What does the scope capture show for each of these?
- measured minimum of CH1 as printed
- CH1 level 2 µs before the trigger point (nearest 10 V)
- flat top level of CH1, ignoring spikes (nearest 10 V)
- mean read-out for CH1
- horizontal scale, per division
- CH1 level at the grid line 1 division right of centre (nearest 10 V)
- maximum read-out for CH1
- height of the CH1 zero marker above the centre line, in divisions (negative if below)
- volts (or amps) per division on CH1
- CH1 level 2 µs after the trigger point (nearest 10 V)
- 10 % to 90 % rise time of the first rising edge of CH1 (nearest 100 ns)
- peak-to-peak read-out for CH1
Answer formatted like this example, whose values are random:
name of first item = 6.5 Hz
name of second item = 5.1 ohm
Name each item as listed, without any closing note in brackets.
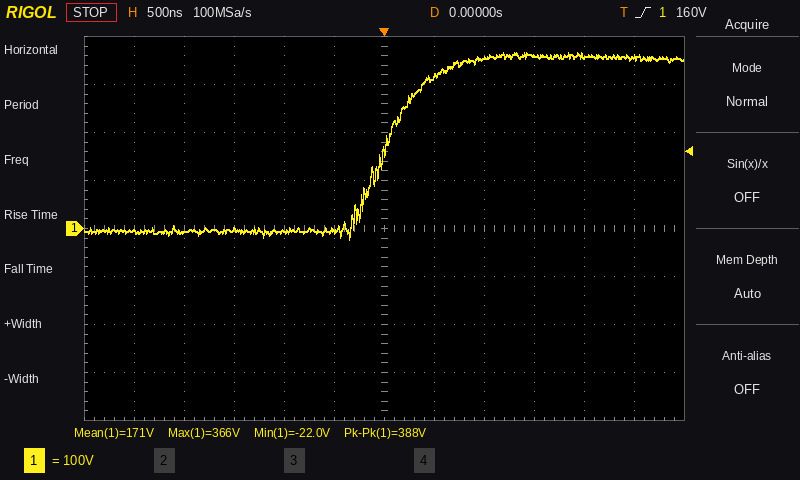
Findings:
measured minimum of CH1 as printed = -22.0 V
CH1 level 2 µs before the trigger point = -10 V
flat top level of CH1, ignoring spikes = 360 V
mean read-out for CH1 = 171 V
horizontal scale, per division = 500 ns
CH1 level at the grid line 1 division right of centre = 320 V
maximum read-out for CH1 = 366 V
height of the CH1 zero marker above the centre line, in divisions = 0.0 div
volts (or amps) per division on CH1 = 100 V
CH1 level 2 µs after the trigger point = 360 V
10 % to 90 % rise time of the first rising edge of CH1 = 800 ns
peak-to-peak read-out for CH1 = 388 V
